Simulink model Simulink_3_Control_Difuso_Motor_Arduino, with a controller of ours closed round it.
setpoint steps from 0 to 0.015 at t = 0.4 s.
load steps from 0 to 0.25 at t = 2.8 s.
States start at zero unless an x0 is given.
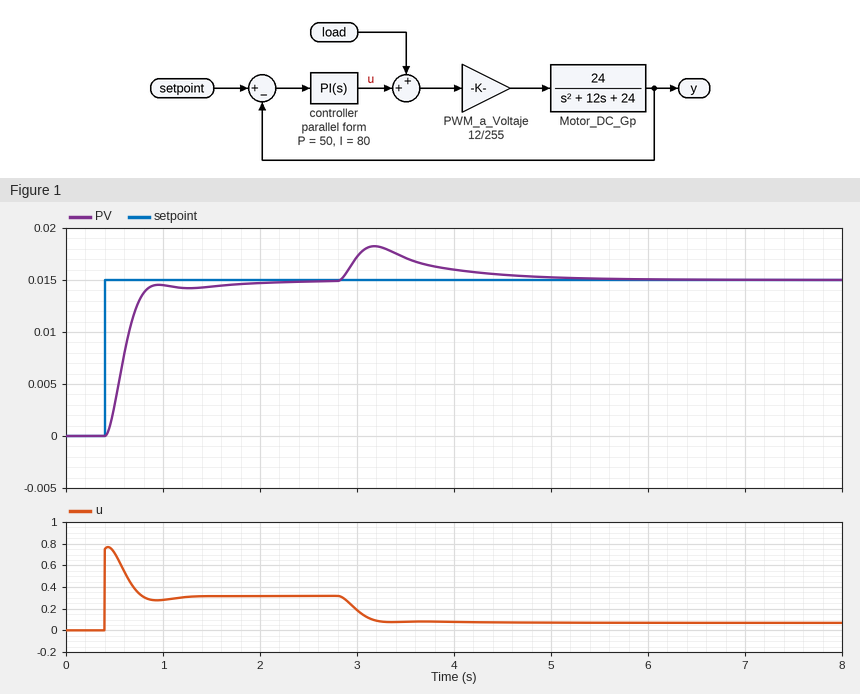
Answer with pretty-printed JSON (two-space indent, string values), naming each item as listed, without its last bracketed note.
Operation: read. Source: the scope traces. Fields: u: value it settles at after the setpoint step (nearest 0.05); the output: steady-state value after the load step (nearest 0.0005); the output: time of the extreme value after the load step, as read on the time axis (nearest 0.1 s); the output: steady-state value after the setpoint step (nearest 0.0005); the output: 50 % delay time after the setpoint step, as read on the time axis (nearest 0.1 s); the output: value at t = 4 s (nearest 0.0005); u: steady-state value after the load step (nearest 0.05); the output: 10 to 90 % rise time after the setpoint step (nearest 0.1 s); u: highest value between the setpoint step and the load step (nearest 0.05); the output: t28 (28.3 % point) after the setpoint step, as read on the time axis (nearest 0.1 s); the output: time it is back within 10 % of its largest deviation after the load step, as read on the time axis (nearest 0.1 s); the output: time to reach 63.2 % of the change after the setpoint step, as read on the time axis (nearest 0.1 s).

{
  "u: value it settles at after the setpoint step": "0.30",
  "the output: steady-state value after the load step": "0.0150",
  "the output: time of the extreme value after the load step, as read on the time axis": "3.2 s",
  "the output: steady-state value after the setpoint step": "0.0150",
  "the output: 50 % delay time after the setpoint step, as read on the time axis": "0.6 s",
  "the output: value at t = 4 s": "0.0160",
  "u: steady-state value after the load step": "0.05",
  "the output: 10 to 90 % rise time after the setpoint step": "0.3 s",
  "u: highest value between the setpoint step and the load step": "0.75",
  "the output: t28 (28.3 % point) after the setpoint step, as read on the time axis": "0.5 s",
  "the output: time it is back within 10 % of its largest deviation after the load step, as read on the time axis": "4.8 s",
  "the output: time to reach 63.2 % of the change after the setpoint step, as read on the time axis": "0.6 s"
}
